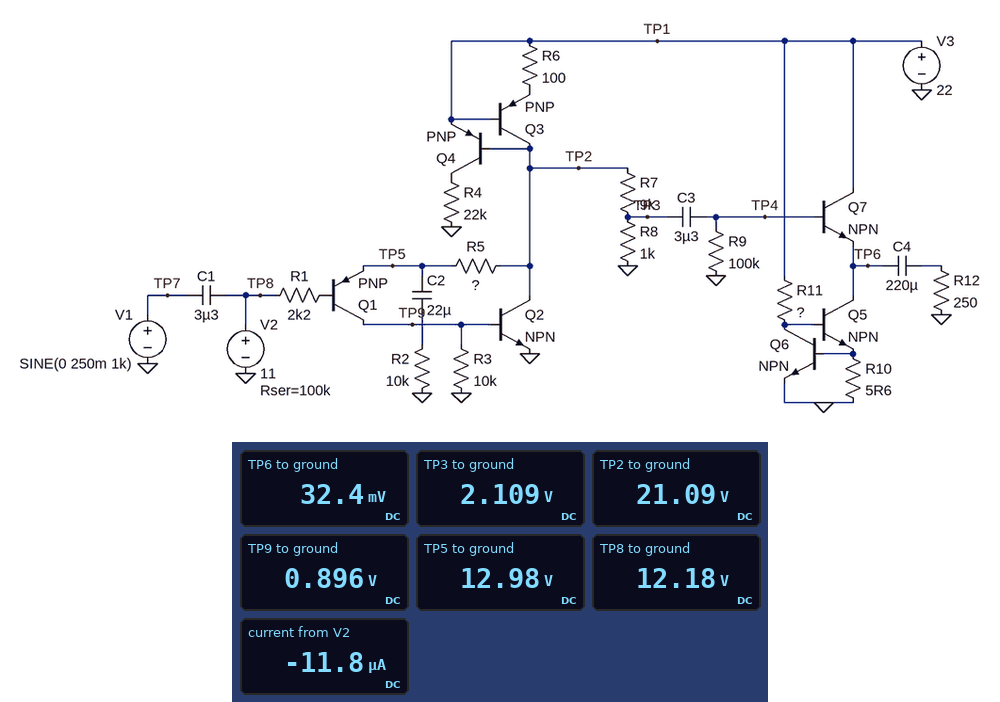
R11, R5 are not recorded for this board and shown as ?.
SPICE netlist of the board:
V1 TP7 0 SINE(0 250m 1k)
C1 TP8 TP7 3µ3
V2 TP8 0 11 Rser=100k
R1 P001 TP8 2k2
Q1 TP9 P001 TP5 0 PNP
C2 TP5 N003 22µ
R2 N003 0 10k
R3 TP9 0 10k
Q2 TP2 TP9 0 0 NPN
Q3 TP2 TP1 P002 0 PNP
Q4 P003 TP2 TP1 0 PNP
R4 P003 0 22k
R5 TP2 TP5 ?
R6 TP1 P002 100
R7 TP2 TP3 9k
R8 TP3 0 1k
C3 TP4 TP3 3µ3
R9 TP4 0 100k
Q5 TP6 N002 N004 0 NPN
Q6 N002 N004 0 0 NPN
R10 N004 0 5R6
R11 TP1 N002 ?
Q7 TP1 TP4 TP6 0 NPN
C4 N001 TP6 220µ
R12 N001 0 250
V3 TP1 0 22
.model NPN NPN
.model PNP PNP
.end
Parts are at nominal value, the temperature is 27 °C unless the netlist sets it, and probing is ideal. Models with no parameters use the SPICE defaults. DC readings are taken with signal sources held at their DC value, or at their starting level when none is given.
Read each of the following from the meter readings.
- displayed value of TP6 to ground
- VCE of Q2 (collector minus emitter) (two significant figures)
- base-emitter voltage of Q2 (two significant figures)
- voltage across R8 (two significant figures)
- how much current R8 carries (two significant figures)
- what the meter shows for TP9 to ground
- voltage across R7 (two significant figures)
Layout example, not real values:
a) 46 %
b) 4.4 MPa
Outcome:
a) 32.4 mV
b) 21 V
c) 900 mV
d) 2.1 V
e) 2.1 mA
f) 0.896 V
g) 19 V
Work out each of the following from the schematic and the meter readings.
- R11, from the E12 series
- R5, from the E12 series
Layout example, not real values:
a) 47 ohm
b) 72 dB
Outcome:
a) 8.2 kΩ
b) 6.8 kΩ
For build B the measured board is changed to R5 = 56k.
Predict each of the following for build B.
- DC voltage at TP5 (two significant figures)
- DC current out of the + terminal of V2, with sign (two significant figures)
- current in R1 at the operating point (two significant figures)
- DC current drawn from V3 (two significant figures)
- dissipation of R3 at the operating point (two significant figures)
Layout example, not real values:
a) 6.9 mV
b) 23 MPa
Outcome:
a) 12 V
b) -1.6 µA
c) 1.6 µA
d) 14 mA
e) 69 µW
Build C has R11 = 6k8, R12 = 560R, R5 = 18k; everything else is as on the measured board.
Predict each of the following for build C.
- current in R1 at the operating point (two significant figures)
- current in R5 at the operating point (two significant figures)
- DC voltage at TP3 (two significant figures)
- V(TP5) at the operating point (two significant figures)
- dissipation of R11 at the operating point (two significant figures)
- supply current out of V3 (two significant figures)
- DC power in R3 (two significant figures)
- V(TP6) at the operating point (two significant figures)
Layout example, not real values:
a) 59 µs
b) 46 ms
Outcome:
a) 4.9 µA
b) 490 µA
c) 2.1 V
d) 12 V
e) 66 mW
f) 47 mA
g) 76 µW
h) 35 mV
